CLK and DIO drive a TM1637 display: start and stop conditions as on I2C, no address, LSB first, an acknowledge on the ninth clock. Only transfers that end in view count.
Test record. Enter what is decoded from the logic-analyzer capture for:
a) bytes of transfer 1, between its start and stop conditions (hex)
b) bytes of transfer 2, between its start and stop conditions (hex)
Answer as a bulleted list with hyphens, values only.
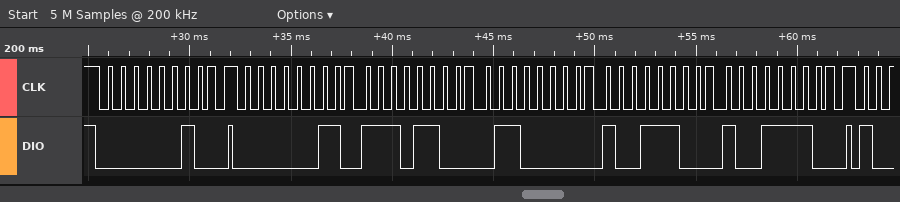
- 40
- C0 37 06 39 79
